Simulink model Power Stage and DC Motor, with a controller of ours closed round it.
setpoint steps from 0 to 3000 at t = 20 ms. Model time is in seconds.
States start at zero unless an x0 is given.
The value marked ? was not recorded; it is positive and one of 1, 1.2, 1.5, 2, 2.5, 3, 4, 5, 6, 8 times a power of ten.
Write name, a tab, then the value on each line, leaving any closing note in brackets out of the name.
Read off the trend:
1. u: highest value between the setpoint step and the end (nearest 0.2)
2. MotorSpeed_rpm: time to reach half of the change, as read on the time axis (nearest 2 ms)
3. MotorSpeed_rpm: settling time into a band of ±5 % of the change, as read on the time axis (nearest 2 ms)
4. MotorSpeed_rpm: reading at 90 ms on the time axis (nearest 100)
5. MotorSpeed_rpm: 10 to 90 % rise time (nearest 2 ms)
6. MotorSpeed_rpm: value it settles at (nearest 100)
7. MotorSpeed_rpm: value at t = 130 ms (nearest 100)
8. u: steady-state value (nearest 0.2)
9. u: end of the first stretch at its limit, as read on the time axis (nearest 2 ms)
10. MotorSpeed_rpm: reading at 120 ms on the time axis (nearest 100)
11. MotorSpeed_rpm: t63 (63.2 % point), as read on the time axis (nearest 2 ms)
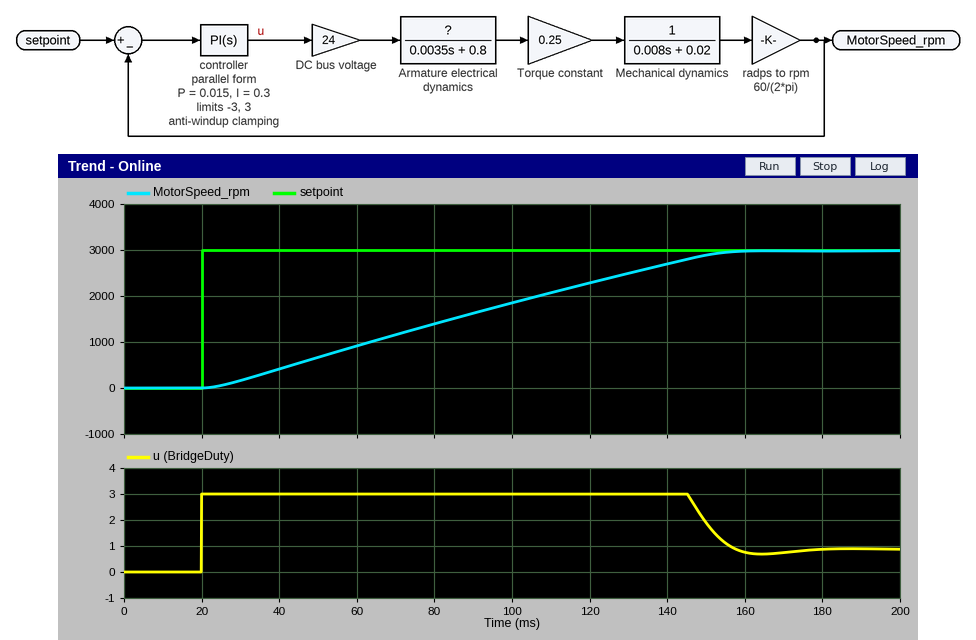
u: highest value between the setpoint step and the end	3.0
MotorSpeed_rpm: time to reach half of the change, as read on the time axis	84 ms
MotorSpeed_rpm: settling time into a band of ±5 % of the change, as read on the time axis	148 ms
MotorSpeed_rpm: reading at 90 ms on the time axis	1600
MotorSpeed_rpm: 10 to 90 % rise time	104 ms
MotorSpeed_rpm: value it settles at	3000
MotorSpeed_rpm: value at t = 130 ms	2500
u: steady-state value	0.8
u: end of the first stretch at its limit, as read on the time axis	146 ms
MotorSpeed_rpm: reading at 120 ms on the time axis	2300
MotorSpeed_rpm: t63 (63.2 % point), as read on the time axis	102 ms
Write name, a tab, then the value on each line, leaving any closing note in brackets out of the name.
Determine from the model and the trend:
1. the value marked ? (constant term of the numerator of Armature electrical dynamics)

the value marked ?	1
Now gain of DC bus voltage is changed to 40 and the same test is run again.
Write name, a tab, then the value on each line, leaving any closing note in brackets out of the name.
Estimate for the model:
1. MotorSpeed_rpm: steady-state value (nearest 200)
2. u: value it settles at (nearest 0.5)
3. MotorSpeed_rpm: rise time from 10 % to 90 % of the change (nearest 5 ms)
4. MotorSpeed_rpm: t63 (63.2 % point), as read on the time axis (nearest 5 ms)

MotorSpeed_rpm: steady-state value	3000
u: value it settles at	0.5
MotorSpeed_rpm: rise time from 10 % to 90 % of the change	60 ms
MotorSpeed_rpm: t63 (63.2 % point), as read on the time axis	70 ms
